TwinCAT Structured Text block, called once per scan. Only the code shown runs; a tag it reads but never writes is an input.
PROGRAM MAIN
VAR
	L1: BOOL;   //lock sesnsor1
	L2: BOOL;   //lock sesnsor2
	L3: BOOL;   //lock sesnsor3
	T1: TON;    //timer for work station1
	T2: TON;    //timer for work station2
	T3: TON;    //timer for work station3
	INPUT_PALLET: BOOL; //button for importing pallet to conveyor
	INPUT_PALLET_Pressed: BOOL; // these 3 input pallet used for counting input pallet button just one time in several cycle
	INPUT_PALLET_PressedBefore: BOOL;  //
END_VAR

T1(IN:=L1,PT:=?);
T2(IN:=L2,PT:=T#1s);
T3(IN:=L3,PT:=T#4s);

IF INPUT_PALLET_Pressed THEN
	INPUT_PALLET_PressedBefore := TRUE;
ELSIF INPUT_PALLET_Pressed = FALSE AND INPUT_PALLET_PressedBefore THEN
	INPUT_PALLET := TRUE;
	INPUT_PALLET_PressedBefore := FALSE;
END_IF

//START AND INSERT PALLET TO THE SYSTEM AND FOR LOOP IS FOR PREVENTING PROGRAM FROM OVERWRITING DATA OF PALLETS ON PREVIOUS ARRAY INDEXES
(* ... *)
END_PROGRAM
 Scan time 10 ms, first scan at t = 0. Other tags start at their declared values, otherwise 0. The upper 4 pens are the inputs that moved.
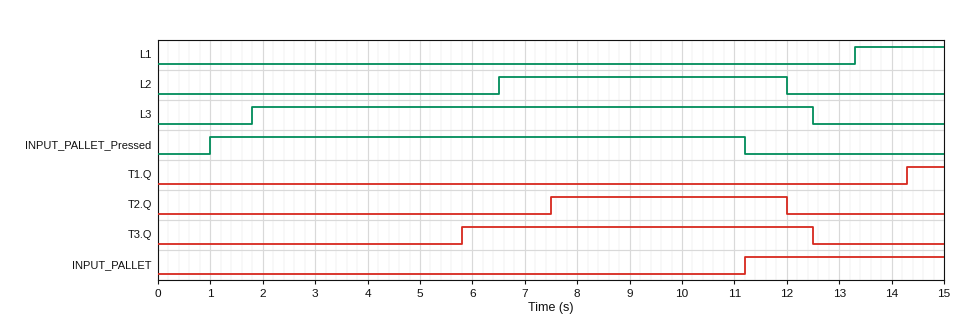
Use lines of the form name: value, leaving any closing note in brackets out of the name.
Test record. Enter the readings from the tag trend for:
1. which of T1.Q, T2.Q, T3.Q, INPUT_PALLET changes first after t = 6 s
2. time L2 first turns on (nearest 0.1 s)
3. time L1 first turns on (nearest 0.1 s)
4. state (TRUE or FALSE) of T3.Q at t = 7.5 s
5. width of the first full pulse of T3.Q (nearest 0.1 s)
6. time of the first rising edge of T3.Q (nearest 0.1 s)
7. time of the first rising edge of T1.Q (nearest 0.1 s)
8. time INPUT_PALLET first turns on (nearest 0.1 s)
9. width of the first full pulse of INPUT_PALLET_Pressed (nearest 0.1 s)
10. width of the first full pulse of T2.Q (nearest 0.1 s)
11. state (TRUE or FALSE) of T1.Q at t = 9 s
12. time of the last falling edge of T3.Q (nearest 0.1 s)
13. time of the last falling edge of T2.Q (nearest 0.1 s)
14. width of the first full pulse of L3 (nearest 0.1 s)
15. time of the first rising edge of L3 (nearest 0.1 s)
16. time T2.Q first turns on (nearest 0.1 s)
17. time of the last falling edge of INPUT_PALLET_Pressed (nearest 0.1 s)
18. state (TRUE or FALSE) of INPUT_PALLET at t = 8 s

which of T1.Q, T2.Q, T3.Q, INPUT_PALLET changes first after t = 6 s: T2.Q
time L2 first turns on: 6.5 s
time L1 first turns on: 13.3 s
state (TRUE or FALSE) of T3.Q at t = 7.5 s: TRUE
width of the first full pulse of T3.Q: 6.7 s
time of the first rising edge of T3.Q: 5.8 s
time of the first rising edge of T1.Q: 14.3 s
time INPUT_PALLET first turns on: 11.2 s
width of the first full pulse of INPUT_PALLET_Pressed: 10.2 s
width of the first full pulse of T2.Q: 4.5 s
state (TRUE or FALSE) of T1.Q at t = 9 s: FALSE
time of the last falling edge of T3.Q: 12.5 s
time of the last falling edge of T2.Q: 12.0 s
width of the first full pulse of L3: 10.7 s
time of the first rising edge of L3: 1.8 s
time T2.Q first turns on: 7.5 s
time of the last falling edge of INPUT_PALLET_Pressed: 11.2 s
state (TRUE or FALSE) of INPUT_PALLET at t = 8 s: FALSE
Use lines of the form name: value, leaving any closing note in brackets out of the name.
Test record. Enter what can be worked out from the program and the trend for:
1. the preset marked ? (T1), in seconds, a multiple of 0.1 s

the preset marked ? (T1), in seconds, a multiple of 0.1 s: 1.0 s
